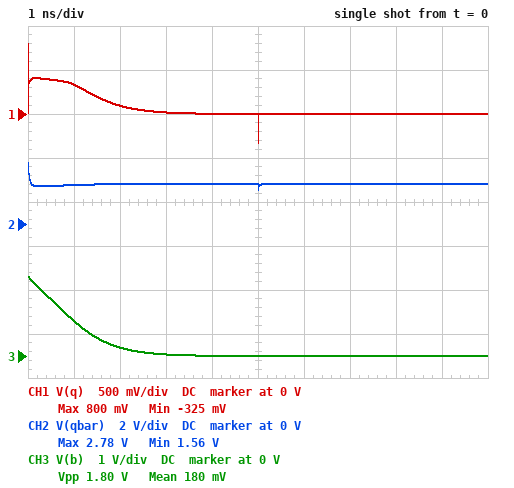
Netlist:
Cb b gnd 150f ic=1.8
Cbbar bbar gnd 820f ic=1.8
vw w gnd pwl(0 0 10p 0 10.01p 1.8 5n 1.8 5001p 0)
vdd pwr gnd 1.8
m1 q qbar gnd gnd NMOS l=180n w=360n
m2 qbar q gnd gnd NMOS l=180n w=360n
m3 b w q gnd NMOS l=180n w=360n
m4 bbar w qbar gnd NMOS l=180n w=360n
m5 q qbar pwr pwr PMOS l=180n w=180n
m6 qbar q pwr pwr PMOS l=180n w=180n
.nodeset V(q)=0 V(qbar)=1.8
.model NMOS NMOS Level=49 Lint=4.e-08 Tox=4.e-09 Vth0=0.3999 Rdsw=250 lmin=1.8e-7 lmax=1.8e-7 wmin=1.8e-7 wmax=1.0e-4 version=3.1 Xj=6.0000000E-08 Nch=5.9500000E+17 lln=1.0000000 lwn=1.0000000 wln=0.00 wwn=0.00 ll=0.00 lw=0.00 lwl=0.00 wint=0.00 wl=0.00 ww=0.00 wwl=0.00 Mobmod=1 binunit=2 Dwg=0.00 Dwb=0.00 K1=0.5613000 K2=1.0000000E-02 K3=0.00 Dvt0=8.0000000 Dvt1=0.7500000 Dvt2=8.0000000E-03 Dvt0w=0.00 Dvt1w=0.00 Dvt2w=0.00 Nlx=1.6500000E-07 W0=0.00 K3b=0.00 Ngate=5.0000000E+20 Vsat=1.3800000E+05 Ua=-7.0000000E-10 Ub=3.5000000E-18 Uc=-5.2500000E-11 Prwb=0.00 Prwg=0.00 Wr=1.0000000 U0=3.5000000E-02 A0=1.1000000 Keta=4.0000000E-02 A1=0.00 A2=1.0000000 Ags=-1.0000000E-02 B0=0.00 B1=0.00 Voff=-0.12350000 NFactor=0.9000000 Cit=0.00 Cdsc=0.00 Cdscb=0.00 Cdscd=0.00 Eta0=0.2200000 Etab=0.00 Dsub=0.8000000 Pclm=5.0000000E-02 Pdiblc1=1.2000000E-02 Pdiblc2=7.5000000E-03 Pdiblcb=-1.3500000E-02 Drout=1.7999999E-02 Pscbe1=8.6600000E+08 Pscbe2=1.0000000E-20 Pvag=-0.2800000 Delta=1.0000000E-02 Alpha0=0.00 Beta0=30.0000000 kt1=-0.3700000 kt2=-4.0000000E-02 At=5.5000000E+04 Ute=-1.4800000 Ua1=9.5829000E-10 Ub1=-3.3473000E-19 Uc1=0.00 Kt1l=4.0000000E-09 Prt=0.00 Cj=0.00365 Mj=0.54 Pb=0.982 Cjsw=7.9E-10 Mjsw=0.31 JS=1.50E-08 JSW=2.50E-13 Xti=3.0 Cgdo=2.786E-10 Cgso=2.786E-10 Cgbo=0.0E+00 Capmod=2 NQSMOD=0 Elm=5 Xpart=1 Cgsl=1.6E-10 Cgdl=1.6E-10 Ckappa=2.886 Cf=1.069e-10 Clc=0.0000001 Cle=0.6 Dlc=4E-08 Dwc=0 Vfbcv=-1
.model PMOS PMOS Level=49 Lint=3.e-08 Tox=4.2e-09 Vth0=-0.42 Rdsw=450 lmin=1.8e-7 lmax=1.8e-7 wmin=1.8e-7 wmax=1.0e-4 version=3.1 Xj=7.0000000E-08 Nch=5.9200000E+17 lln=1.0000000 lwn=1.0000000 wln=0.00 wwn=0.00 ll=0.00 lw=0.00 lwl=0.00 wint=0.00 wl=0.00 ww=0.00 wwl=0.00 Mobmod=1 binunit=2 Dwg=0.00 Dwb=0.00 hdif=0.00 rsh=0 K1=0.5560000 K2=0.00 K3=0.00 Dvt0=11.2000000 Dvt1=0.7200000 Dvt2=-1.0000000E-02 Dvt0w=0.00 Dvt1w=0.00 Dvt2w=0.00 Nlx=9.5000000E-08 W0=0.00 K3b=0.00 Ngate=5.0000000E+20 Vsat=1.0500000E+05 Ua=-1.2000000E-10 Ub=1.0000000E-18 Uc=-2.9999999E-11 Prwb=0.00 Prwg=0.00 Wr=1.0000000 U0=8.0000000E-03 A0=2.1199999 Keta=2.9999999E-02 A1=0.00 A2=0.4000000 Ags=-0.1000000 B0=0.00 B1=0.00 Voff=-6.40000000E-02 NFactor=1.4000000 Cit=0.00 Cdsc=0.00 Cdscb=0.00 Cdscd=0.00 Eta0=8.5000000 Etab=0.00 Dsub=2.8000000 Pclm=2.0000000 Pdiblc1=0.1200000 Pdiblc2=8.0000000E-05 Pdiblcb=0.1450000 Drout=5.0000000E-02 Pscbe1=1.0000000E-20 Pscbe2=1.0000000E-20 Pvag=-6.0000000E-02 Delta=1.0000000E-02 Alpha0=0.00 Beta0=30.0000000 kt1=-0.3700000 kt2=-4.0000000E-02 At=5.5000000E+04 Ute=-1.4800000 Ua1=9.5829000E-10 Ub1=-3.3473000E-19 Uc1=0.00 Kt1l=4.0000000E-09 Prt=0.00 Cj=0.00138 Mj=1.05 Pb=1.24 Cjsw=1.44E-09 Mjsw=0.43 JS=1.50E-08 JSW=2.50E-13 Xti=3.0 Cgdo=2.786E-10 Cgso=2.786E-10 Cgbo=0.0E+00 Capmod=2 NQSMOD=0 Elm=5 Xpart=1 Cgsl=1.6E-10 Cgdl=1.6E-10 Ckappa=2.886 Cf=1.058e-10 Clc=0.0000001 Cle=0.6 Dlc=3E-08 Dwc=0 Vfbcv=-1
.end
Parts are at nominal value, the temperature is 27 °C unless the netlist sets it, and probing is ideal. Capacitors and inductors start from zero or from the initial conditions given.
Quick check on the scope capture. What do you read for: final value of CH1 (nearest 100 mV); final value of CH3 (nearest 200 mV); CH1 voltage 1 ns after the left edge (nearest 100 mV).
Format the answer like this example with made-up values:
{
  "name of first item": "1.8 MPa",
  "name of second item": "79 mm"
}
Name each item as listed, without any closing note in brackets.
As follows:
{
  "final value of CH1": "0 V",
  "final value of CH3": "0 V",
  "CH1 voltage 1 ns after the left edge": "300 mV"
}
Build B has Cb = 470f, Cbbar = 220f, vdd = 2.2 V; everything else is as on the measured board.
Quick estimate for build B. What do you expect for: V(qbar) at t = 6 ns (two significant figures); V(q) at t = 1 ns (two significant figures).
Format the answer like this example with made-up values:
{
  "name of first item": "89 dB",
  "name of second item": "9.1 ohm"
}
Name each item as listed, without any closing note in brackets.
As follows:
{
  "V(qbar) at t = 6 ns": "2.2 V",
  "V(q) at t = 1 ns": "360 mV"
}
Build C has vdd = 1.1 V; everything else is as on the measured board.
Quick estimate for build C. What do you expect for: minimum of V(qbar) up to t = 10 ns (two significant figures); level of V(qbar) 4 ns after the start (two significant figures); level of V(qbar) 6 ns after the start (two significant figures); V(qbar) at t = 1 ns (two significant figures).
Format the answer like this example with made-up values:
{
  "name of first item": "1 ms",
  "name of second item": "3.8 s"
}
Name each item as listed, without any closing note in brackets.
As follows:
{
  "minimum of V(qbar) up to t = 10 ns": "870 mV",
  "level of V(qbar) 4 ns after the start": "1.2 V",
  "level of V(qbar) 6 ns after the start": "1.1 V",
  "V(qbar) at t = 1 ns": "910 mV"
}
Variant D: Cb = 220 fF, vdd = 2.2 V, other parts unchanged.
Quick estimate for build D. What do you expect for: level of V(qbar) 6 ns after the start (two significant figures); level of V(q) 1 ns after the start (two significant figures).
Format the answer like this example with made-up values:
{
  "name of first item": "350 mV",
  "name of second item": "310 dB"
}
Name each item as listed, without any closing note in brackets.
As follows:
{
  "level of V(qbar) 6 ns after the start": "2.2 V",
  "level of V(q) 1 ns after the start": "340 mV"
}
